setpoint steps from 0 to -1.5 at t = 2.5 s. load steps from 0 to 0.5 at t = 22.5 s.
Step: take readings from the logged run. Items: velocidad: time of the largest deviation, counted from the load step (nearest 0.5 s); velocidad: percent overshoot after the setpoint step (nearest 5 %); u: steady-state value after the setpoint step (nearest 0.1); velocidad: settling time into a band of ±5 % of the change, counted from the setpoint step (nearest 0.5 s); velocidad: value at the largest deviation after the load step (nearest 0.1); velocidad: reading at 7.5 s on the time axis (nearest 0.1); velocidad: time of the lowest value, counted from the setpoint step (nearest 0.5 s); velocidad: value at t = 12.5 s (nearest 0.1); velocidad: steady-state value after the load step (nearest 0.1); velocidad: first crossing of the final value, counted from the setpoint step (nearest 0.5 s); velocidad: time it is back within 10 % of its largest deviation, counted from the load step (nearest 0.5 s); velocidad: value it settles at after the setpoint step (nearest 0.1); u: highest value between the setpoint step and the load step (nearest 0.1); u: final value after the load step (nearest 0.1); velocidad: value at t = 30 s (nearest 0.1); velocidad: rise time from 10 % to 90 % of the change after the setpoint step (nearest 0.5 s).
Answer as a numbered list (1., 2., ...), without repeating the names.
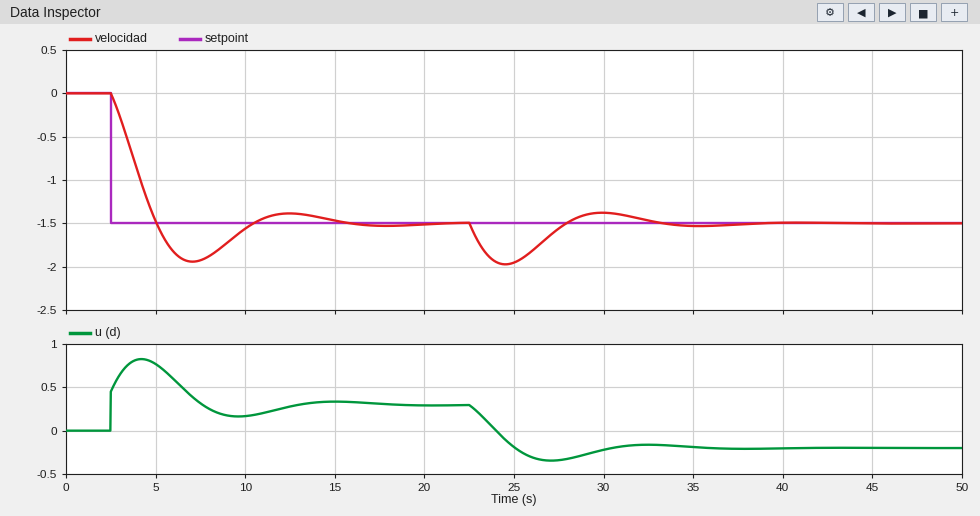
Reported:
1. 2.0 s
2. 30 %
3. 0.3
4. 11.5 s
5. -2.0
6. -1.9
7. 4.5 s
8. -1.4
9. -1.5
10. 2.5 s
11. 9.5 s
12. -1.5
13. 0.8
14. -0.2
15. -1.4
16. 2.0 s
